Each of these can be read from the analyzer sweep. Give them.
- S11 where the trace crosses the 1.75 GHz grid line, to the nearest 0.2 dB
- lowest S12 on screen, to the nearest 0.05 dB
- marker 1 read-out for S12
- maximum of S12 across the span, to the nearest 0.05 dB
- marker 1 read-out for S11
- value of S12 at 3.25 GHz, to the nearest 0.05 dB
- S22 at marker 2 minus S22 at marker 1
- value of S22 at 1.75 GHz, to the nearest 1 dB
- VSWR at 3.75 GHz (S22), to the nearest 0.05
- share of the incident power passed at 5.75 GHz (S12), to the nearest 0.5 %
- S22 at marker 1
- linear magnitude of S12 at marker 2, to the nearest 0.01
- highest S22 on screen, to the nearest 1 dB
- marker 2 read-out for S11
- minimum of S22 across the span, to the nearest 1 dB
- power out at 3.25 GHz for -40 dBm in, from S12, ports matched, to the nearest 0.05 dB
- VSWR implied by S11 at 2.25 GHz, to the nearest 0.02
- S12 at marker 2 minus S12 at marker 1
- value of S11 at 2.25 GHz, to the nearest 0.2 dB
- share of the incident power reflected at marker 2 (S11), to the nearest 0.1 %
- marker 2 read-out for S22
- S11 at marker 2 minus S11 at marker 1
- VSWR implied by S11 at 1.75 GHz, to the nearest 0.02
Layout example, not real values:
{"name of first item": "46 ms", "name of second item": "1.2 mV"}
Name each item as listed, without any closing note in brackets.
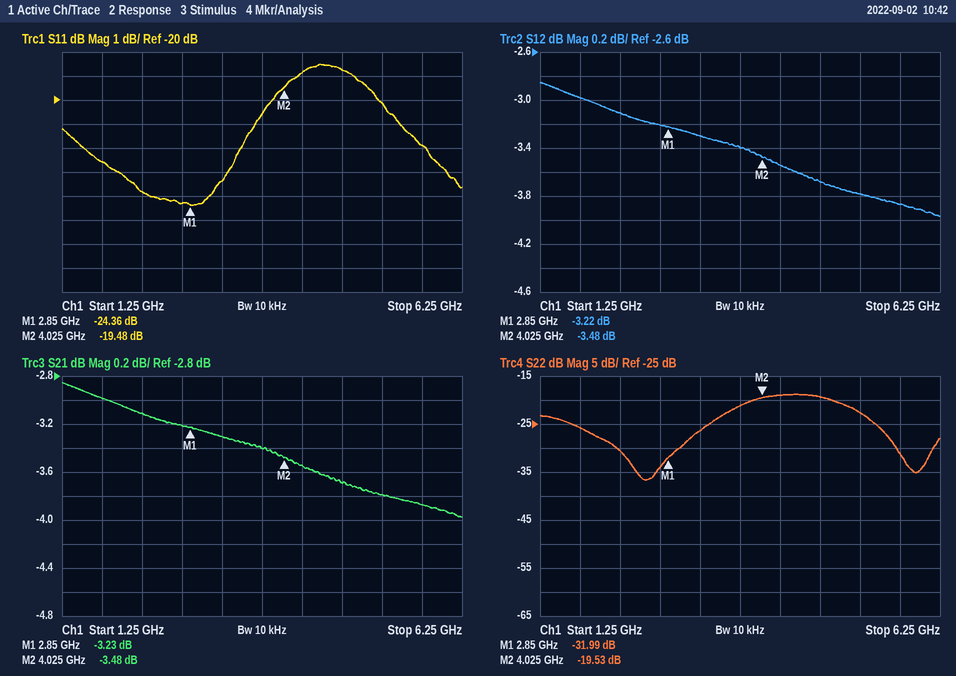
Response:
{"S11 where the trace crosses the 1.75 GHz grid line, to the nearest 0.2 dB": "-22.6 dB", "lowest S12 on screen, to the nearest 0.05 dB": "-3.95 dB", "marker 1 read-out for S12": "-3.22 dB", "maximum of S12 across the span, to the nearest 0.05 dB": "-2.85 dB", "marker 1 read-out for S11": "-24.36 dB", "value of S12 at 3.25 GHz, to the nearest 0.05 dB": "-3.30 dB", "S22 at marker 2 minus S22 at marker 1": "12.46 dB", "value of S22 at 1.75 GHz, to the nearest 1 dB": "-26 dB", "VSWR at 3.75 GHz (S22), to the nearest 0.05": "1.20", "share of the incident power passed at 5.75 GHz (S12), to the nearest 0.5 %": "41.0 %", "S22 at marker 1": "-31.99 dB", "linear magnitude of S12 at marker 2, to the nearest 0.01": "0.67", "highest S22 on screen, to the nearest 1 dB": "-19 dB", "marker 2 read-out for S11": "-19.48 dB", "minimum of S22 across the span, to the nearest 1 dB": "-37 dB", "power out at 3.25 GHz for -40 dBm in, from S12, ports matched, to the nearest 0.05 dB": "-43.30 dBm", "VSWR implied by S11 at 2.25 GHz, to the nearest 0.02": "1.14", "S12 at marker 2 minus S12 at marker 1": "-0.26 dB", "value of S11 at 2.25 GHz, to the nearest 0.2 dB": "-23.8 dB", "share of the incident power reflected at marker 2 (S11), to the nearest 0.1 %": "1.1 %", "marker 2 read-out for S22": "-19.53 dB", "S11 at marker 2 minus S11 at marker 1": "4.88 dB", "VSWR implied by S11 at 1.75 GHz, to the nearest 0.02": "1.16"}
